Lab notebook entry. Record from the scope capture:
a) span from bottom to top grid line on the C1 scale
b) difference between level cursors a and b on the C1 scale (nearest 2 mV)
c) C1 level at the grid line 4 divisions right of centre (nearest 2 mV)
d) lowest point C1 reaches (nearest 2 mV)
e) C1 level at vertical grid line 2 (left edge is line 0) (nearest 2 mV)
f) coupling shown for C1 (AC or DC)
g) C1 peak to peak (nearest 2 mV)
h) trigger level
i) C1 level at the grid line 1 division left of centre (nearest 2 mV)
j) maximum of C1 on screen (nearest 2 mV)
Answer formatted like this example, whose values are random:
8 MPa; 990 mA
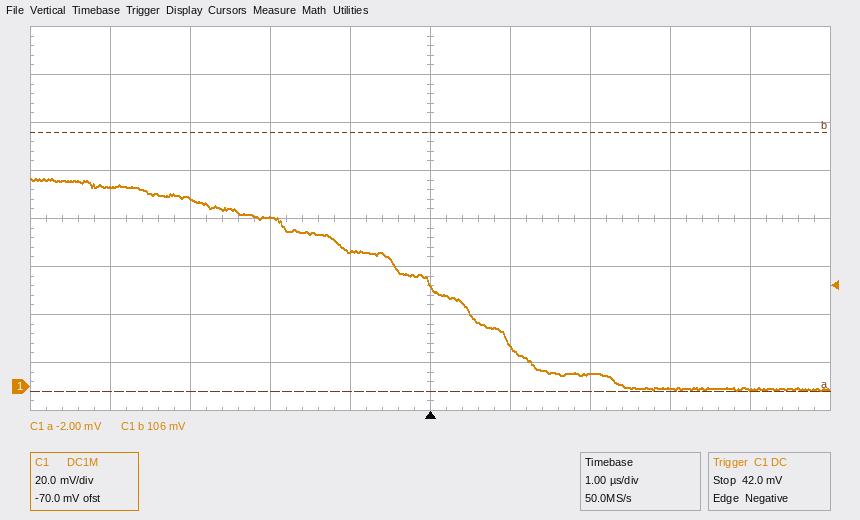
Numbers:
160 mV; 108 mV; -2 mV; -2 mV; 78 mV; DC; 88 mV; 42.0 mV; 56 mV; 86 mV
